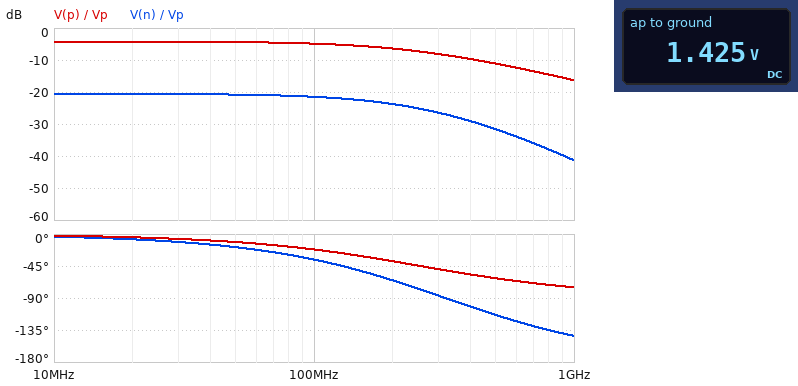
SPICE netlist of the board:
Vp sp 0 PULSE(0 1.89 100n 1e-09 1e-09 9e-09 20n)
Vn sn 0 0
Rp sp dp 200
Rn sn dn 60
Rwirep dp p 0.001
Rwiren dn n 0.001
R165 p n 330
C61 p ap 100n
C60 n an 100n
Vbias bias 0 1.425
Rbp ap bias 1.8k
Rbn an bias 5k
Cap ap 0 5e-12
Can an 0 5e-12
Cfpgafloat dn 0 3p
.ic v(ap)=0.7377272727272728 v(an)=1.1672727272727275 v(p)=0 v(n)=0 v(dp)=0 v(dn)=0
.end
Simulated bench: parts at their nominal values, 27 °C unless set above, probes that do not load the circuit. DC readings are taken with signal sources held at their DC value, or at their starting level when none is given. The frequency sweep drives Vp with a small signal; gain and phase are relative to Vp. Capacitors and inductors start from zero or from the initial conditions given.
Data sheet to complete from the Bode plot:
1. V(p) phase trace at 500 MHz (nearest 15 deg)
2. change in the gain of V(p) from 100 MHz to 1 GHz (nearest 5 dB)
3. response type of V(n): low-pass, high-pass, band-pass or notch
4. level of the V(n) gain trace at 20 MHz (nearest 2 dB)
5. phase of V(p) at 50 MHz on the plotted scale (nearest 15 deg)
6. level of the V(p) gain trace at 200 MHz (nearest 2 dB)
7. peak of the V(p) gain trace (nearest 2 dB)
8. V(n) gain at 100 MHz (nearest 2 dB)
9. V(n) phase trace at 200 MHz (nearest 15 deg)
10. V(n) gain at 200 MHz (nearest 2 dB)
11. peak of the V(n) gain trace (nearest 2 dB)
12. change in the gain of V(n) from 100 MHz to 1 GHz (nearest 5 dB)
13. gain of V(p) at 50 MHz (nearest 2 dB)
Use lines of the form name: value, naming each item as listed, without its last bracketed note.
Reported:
V(p) phase trace at 500 MHz: -60 deg
change in the gain of V(p) from 100 MHz to 1 GHz: -10 dB
response type of V(n): low-pass, high-pass, band-pass or notch: low-pass
level of the V(n) gain trace at 20 MHz: -20 dB
phase of V(p) at 50 MHz on the plotted scale: -15 deg
level of the V(p) gain trace at 200 MHz: -6 dB
peak of the V(p) gain trace: -4 dB
V(n) gain at 100 MHz: -22 dB
V(n) phase trace at 200 MHz: -60 deg
V(n) gain at 200 MHz: -24 dB
peak of the V(n) gain trace: -20 dB
change in the gain of V(n) from 100 MHz to 1 GHz: -20 dB
gain of V(p) at 50 MHz: -4 dB
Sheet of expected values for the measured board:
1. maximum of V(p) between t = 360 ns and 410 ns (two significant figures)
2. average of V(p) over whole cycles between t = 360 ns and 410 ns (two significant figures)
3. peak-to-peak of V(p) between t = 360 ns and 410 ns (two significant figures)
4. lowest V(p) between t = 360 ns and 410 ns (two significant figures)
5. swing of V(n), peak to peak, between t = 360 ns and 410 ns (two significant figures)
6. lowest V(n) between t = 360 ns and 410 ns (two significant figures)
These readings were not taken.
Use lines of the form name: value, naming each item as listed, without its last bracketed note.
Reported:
maximum of V(p) between t = 360 ns and 410 ns: 1.2 V
average of V(p) over whole cycles between t = 360 ns and 410 ns: 630 mV
peak-to-peak of V(p) between t = 360 ns and 410 ns: 1.2 V
lowest V(p) between t = 360 ns and 410 ns: 48 mV
swing of V(n), peak to peak, between t = 360 ns and 410 ns: 180 mV
lowest V(n) between t = 360 ns and 410 ns: 9.9 mV
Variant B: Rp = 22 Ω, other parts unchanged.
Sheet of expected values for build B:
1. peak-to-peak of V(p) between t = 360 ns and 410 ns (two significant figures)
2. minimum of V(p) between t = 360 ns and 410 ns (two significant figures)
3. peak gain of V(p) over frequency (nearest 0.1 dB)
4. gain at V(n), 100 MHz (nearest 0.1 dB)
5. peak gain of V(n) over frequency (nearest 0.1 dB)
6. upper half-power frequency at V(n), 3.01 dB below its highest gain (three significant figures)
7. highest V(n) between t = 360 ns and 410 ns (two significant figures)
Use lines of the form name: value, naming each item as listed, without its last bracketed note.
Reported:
peak-to-peak of V(p) between t = 360 ns and 410 ns: 1.8 V
minimum of V(p) between t = 360 ns and 410 ns: 8.0 mV
peak gain of V(p) over frequency: -0.6 dB
gain at V(n), 100 MHz: -17.2 dB
peak gain of V(n) over frequency: -16.9 dB
upper half-power frequency at V(n), 3.01 dB below its highest gain: 370 MHz
highest V(n) between t = 360 ns and 410 ns: 270 mV
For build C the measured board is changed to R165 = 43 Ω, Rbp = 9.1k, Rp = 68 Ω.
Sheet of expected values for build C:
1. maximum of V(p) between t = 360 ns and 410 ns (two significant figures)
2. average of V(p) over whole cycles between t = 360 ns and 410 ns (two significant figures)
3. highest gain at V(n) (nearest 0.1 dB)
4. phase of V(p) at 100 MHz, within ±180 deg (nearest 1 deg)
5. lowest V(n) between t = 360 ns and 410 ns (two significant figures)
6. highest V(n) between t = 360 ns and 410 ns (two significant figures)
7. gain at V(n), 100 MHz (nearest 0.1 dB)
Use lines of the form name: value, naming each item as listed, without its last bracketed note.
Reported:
maximum of V(p) between t = 360 ns and 410 ns: 1.1 V
average of V(p) over whole cycles between t = 360 ns and 410 ns: 570 mV
highest gain at V(n): -9.2 dB
phase of V(p) at 100 MHz, within ±180 deg: -11 deg
lowest V(n) between t = 360 ns and 410 ns: 3.8 mV
highest V(n) between t = 360 ns and 410 ns: 660 mV
gain at V(n), 100 MHz: -9.5 dB
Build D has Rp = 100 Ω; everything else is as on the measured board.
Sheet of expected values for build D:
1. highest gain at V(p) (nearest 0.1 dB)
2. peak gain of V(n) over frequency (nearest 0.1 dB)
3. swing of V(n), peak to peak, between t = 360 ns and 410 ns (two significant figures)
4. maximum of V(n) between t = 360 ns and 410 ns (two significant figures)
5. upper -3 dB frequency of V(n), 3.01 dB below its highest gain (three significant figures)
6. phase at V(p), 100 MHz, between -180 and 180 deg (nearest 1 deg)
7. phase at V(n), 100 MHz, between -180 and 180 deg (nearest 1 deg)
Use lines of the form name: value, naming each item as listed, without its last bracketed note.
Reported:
highest gain at V(p): -2.4 dB
peak gain of V(n) over frequency: -18.7 dB
swing of V(n), peak to peak, between t = 360 ns and 410 ns: 220 mV
maximum of V(n) between t = 360 ns and 410 ns: 230 mV
upper -3 dB frequency of V(n), 3.01 dB below its highest gain: 255 MHz
phase at V(p), 100 MHz, between -180 and 180 deg: -14 deg
phase at V(n), 100 MHz, between -180 and 180 deg: -28 deg
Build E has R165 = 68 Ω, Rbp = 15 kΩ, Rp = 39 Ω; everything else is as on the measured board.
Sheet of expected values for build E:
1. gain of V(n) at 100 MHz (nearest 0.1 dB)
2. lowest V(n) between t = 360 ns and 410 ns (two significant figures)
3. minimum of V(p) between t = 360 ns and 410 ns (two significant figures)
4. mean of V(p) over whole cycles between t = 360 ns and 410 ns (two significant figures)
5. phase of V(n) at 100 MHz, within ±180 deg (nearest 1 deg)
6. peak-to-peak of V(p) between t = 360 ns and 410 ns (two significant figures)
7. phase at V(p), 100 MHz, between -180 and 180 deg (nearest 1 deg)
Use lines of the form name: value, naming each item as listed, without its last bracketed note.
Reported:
gain of V(n) at 100 MHz: -9.2 dB
lowest V(n) between t = 360 ns and 410 ns: 2.6 mV
minimum of V(p) between t = 360 ns and 410 ns: 2.1 mV
mean of V(p) over whole cycles between t = 360 ns and 410 ns: 720 mV
phase of V(n) at 100 MHz, within ±180 deg: -16 deg
peak-to-peak of V(p) between t = 360 ns and 410 ns: 1.4 V
phase at V(p), 100 MHz, between -180 and 180 deg: -7 deg
